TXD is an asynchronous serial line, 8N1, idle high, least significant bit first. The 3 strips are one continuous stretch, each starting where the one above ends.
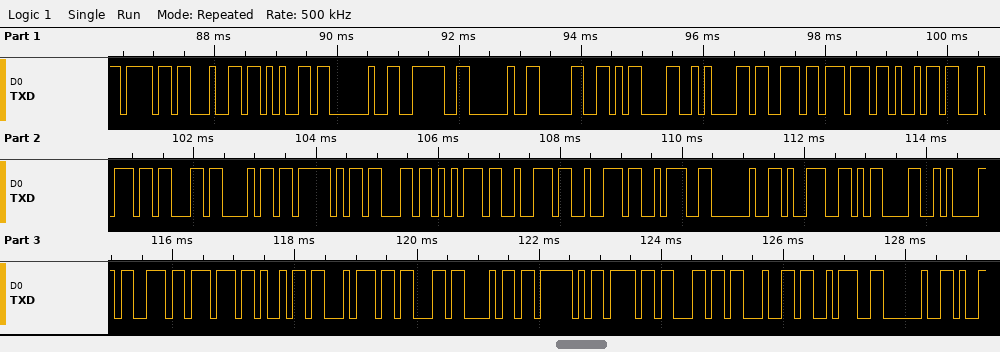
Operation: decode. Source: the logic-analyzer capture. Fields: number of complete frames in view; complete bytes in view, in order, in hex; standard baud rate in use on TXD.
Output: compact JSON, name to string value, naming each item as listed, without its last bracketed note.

{"number of complete frames in view": "37", "complete bytes in view, in order, in hex": "6F 64 65 20 3E 20 30 0D 0A 73 77 69 74 63 68 5F 63 75 72 72 3A 20 39 0D 0A 73 77 69 74 63 68 5F 6F 6C 64 3A 20", "standard baud rate in use on TXD": "9600 baud"}
